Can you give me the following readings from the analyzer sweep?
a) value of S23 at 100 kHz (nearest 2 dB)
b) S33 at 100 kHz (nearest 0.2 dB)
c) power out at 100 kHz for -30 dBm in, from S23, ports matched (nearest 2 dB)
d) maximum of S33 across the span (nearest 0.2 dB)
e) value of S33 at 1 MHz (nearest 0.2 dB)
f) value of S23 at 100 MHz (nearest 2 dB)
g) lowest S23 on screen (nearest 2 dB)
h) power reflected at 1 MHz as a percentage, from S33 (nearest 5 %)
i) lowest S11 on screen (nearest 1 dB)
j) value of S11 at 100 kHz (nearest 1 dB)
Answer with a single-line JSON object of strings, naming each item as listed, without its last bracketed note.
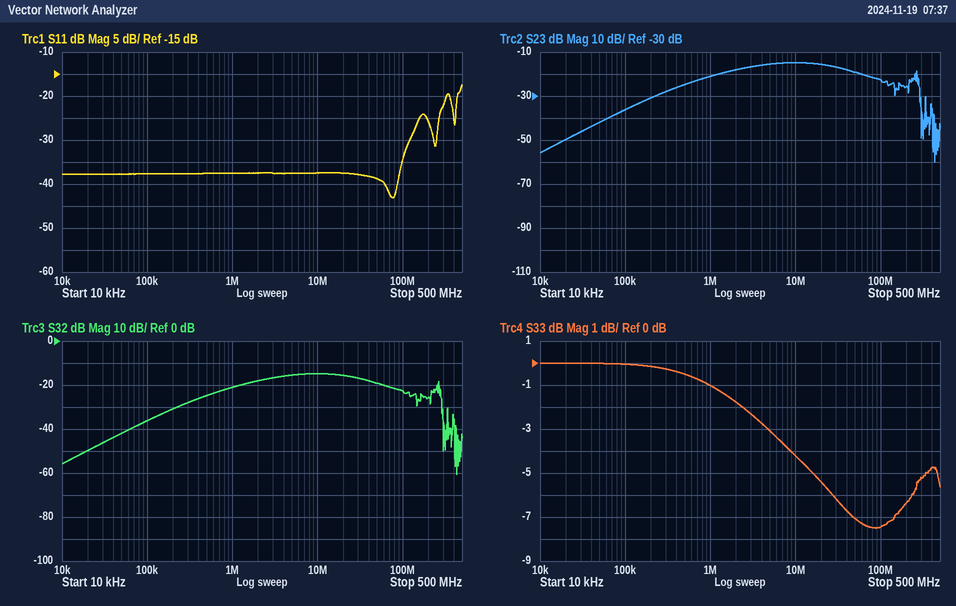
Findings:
{"value of S23 at 100 kHz": "-36 dB", "S33 at 100 kHz": "0.0 dB", "power out at 100 kHz for -30 dBm in, from S23, ports matched": "-66 dBm", "maximum of S33 across the span": "0.0 dB", "value of S33 at 1 MHz": "-1.0 dB", "value of S23 at 100 MHz": "-22 dB", "lowest S23 on screen": "-60 dB", "power reflected at 1 MHz as a percentage, from S33": "80 %", "lowest S11 on screen": "-43 dB", "value of S11 at 100 kHz": "-38 dB"}
